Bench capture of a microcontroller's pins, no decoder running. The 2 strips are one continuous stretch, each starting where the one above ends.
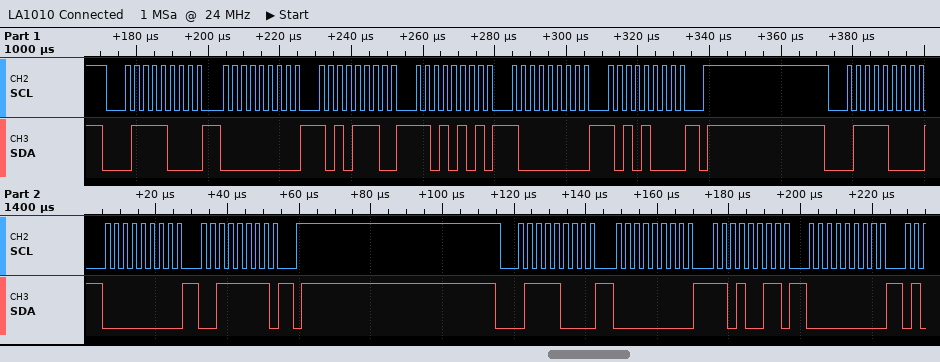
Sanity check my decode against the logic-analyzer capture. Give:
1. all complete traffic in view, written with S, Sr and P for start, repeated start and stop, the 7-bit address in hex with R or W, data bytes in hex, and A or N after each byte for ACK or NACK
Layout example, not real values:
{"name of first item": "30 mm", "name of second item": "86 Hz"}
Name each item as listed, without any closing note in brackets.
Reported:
{"all complete traffic in view, written with S, Sr and P for start, repeated start and stop, the 7-bit address in hex with R or W, data bytes in hex, and A or N after each byte for ACK or NACK": "S 3CW A 00 A AE A D5 A 80 A A8 A P S 3CW A 00 A 3F A P S 3CW A 00 A D3 A 00 A"}
